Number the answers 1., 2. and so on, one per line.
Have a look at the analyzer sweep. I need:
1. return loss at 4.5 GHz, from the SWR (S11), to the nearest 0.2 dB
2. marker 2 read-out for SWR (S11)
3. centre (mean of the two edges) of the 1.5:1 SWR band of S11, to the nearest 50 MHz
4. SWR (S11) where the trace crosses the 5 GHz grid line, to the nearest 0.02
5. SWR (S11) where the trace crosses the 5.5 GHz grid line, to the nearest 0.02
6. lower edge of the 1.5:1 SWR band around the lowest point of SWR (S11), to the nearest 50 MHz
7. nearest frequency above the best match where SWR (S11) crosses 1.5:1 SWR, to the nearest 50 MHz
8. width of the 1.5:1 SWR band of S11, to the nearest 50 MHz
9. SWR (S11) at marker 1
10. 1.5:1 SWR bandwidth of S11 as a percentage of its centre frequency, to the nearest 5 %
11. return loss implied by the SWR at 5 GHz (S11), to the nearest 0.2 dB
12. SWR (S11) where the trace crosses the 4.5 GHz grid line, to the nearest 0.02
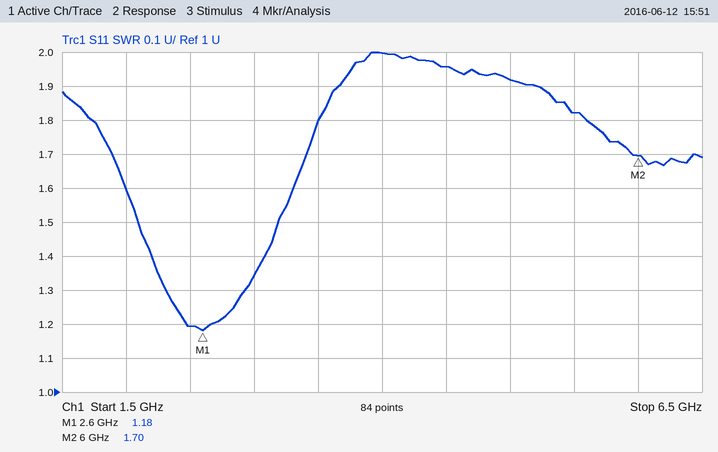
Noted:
1. 9.8 dB
2. 1.70
3. 2.65 GHz
4. 1.92
5. 1.82
6. 2.10 GHz
7. 3.20 GHz
8. 1.10 GHz
9. 1.18
10. 40 %
11. 10.0 dB
12. 1.96
